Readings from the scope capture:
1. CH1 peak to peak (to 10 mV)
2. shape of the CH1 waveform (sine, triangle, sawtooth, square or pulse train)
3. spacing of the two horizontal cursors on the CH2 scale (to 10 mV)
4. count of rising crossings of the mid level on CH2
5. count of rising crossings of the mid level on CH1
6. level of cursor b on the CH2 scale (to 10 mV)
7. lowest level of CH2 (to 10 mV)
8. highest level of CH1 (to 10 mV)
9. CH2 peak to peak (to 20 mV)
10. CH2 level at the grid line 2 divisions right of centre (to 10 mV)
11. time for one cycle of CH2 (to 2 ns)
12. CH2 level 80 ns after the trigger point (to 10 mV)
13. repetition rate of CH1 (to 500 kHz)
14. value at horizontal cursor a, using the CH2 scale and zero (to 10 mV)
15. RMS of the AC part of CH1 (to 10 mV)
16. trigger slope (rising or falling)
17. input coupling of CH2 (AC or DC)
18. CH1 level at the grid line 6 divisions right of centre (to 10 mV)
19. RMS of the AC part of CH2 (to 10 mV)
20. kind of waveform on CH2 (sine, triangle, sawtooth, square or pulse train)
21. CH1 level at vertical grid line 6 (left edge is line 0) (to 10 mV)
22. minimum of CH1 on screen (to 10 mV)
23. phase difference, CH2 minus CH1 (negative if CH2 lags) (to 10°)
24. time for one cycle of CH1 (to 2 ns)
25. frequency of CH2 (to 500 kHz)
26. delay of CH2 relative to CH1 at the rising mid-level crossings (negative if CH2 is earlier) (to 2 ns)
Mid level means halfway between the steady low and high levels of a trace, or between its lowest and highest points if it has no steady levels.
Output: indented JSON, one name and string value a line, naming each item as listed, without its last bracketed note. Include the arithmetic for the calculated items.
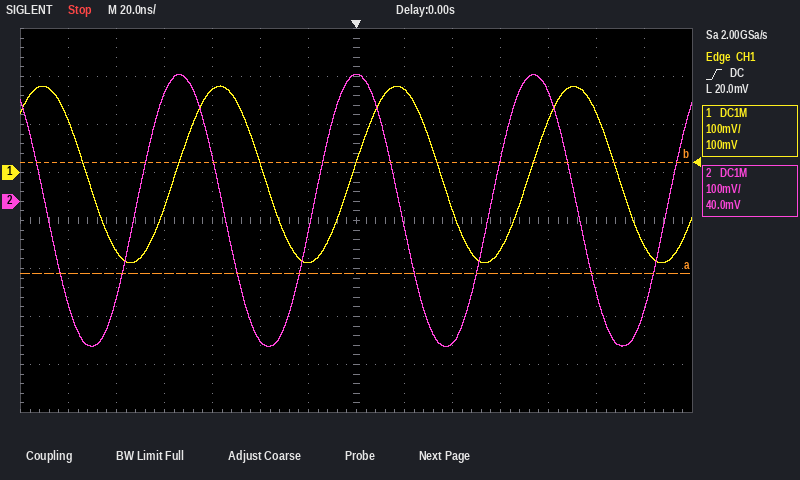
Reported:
{
  "CH1 peak to peak": "180 mV − (-190 mV) = 370 mV",
  "shape of the CH1 waveform": "sine",
  "spacing of the two horizontal cursors on the CH2 scale": "230 mV",
  "count of rising crossings of the mid level on CH2": "4",
  "count of rising crossings of the mid level on CH1": "3",
  "level of cursor b on the CH2 scale": "80 mV",
  "lowest level of CH2": "-300 mV",
  "highest level of CH1": "180 mV",
  "CH2 peak to peak": "560 mV",
  "CH2 level at the grid line 2 divisions right of centre": "-300 mV",
  "time for one cycle of CH2": "74 ns",
  "CH2 level 80 ns after the trigger point": "230 mV",
  "repetition rate of CH1": "1 / 74 ns ≈ 13.5 MHz",
  "value at horizontal cursor a, using the CH2 scale and zero": "-150 mV",
  "RMS of the AC part of CH1": "370 mV / (2√2) ≈ 131 mV, so 130 mV to the nearest 10 mV",
  "trigger slope": "rising",
  "input coupling of CH2": "DC",
  "CH1 level at the grid line 6 divisions right of centre": "-150 mV",
  "RMS of the AC part of CH2": "560 mV / (2√2) ≈ 198 mV, so 200 mV to the nearest 10 mV",
  "kind of waveform on CH2": "sine",
  "CH1 level at vertical grid line 6 (left edge is line 0)": "-190 mV",
  "minimum of CH1 on screen": "-190 mV",
  "phase difference, CH2 minus CH1 (negative if CH2 lags)": "−360° × (-16 ns) / 74 ns ≈ +77.8°, so +80° to the nearest 10°",
  "time for one cycle of CH1": "74 ns",
  "frequency of CH2": "1 / 74 ns ≈ 13.5 MHz",
  "delay of CH2 relative to CH1 at the rising mid-level crossings (negative if CH2 is earlier)": "-16 ns"
}
